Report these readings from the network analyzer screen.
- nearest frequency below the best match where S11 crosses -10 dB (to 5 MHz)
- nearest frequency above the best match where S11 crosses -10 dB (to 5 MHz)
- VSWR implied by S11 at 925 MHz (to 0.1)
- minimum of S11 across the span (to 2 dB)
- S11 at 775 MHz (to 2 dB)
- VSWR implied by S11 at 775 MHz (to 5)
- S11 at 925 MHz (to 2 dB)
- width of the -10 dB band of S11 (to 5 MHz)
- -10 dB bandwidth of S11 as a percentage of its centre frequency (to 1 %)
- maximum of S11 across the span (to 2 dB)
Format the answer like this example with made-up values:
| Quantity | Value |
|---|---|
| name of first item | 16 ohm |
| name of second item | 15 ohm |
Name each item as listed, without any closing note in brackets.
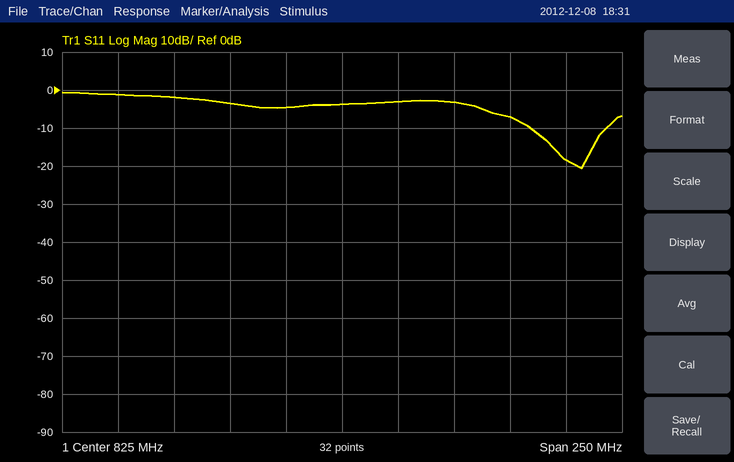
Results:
| Quantity | Value |
|---|---|
| nearest frequency below the best match where S11 crosses -10 dB | 910 MHz |
| nearest frequency above the best match where S11 crosses -10 dB | 945 MHz |
| VSWR implied by S11 at 925 MHz | 1.3 |
| minimum of S11 across the span | -20 dB |
| S11 at 775 MHz | -4 dB |
| VSWR implied by S11 at 775 MHz | 5 |
| S11 at 925 MHz | -18 dB |
| width of the -10 dB band of S11 | 35 MHz |
| -10 dB bandwidth of S11 as a percentage of its centre frequency | 4 % |
| maximum of S11 across the span | 0 dB |
